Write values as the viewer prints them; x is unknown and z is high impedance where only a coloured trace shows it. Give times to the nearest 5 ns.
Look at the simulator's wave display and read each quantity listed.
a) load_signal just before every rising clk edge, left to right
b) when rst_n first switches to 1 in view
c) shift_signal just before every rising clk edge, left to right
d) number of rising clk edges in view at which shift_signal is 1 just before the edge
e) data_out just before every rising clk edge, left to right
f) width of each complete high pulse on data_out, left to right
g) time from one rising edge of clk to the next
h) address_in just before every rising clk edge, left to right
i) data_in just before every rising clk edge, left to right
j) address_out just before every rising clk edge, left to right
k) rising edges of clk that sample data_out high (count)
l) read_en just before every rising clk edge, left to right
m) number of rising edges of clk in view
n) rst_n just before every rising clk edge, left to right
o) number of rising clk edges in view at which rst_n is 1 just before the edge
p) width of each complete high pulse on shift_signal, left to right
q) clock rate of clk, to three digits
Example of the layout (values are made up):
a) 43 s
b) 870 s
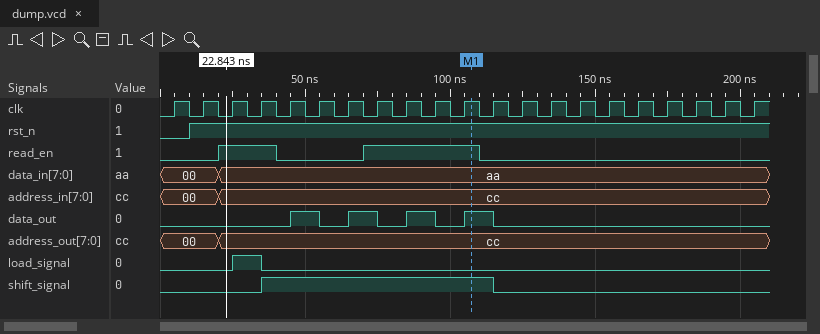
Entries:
a) 0 0 0 1 0 0 0 0 0 0 0 0 0 0 0 0 0 0 0 0 0
b) 10 ns
c) 0 0 0 0 1 1 1 1 1 1 1 1 0 0 0 0 0 0 0 0 0
d) 8
e) 0 0 0 0 0 1 0 1 0 1 0 1 0 0 0 0 0 0 0 0 0
f) 10 ns, 10 ns, 10 ns, 10 ns
g) 10 ns
h) 00, 00, cc, cc, cc, cc, cc, cc, cc, cc, cc, cc, cc, cc, cc, cc, cc, cc, cc, cc, cc
i) 00, 00, aa, aa, aa, aa, aa, aa, aa, aa, aa, aa, aa, aa, aa, aa, aa, aa, aa, aa, aa
j) 00, 00, cc, cc, cc, cc, cc, cc, cc, cc, cc, cc, cc, cc, cc, cc, cc, cc, cc, cc, cc
k) 4
l) 0 0 1 1 0 0 0 1 1 1 1 0 0 0 0 0 0 0 0 0 0
m) 21
n) 0 1 1 1 1 1 1 1 1 1 1 1 1 1 1 1 1 1 1 1 1
o) 20
p) 80 ns
q) 100 MHz
